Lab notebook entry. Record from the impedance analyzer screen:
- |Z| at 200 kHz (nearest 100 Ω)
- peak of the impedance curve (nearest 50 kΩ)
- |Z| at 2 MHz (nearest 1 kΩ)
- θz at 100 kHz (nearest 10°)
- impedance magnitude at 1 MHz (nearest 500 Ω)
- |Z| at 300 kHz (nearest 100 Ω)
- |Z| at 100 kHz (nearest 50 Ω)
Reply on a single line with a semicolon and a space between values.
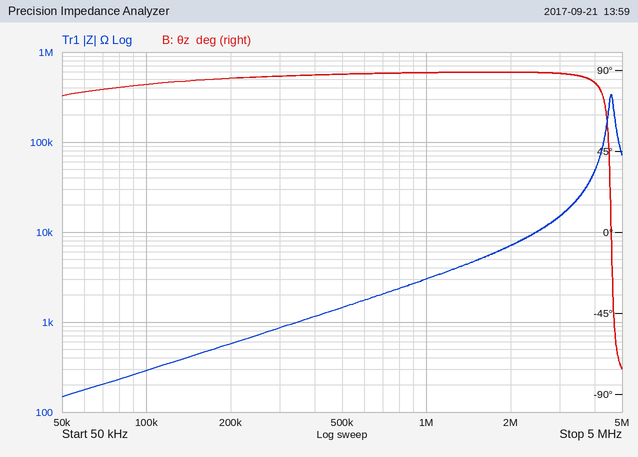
600 Ω; 350 kΩ; 7 kΩ; 80°; 3.0 kΩ; 900 Ω; 300 Ω
